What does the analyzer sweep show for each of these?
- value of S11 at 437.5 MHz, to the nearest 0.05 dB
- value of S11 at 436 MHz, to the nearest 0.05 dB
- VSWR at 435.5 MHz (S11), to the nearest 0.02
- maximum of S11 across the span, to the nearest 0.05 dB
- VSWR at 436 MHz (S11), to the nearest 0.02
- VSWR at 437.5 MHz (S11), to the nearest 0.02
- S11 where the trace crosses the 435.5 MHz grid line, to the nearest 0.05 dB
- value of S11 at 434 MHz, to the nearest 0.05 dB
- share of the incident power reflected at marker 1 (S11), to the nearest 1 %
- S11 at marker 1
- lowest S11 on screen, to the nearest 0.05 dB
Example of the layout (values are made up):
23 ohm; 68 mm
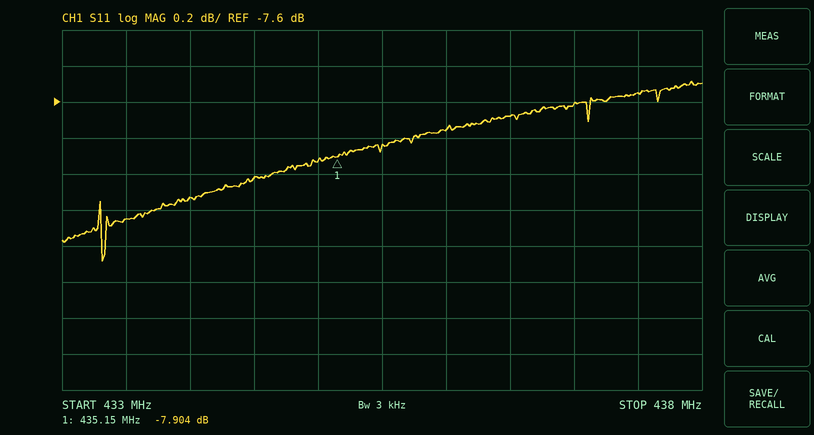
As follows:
-7.55 dB; -7.75 dB; 2.36; -7.50 dB; 2.38; 2.44; -7.85 dB; -8.15 dB; 16 %; -7.904 dB; -8.50 dB
